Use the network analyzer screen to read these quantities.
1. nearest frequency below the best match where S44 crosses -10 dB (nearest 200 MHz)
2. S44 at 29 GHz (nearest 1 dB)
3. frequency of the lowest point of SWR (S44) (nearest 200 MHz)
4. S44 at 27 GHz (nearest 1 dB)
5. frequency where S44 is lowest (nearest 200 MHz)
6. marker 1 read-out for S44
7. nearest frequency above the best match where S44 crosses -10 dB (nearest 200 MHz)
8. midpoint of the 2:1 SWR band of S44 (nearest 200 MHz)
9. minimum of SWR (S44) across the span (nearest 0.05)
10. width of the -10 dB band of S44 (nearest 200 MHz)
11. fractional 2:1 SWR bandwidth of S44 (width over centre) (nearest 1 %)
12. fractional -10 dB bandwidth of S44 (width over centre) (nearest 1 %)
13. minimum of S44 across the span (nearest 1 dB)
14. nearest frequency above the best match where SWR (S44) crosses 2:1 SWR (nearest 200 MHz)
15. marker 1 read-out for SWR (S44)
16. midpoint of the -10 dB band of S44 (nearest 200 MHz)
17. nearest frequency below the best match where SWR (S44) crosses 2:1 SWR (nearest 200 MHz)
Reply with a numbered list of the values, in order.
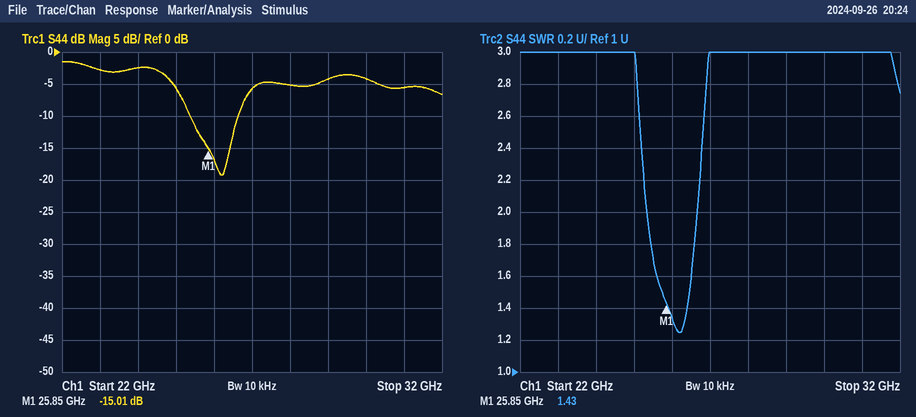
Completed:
1. 25.4 GHz
2. -4 dB
3. 26.2 GHz
4. -6 dB
5. 26.2 GHz
6. -15.01 dB
7. 26.6 GHz
8. 26.0 GHz
9. 1.25
10. 1.2 GHz
11. 5 %
12. 5 %
13. -19 dB
14. 26.6 GHz
15. 1.43
16. 26.0 GHz
17. 25.4 GHz
